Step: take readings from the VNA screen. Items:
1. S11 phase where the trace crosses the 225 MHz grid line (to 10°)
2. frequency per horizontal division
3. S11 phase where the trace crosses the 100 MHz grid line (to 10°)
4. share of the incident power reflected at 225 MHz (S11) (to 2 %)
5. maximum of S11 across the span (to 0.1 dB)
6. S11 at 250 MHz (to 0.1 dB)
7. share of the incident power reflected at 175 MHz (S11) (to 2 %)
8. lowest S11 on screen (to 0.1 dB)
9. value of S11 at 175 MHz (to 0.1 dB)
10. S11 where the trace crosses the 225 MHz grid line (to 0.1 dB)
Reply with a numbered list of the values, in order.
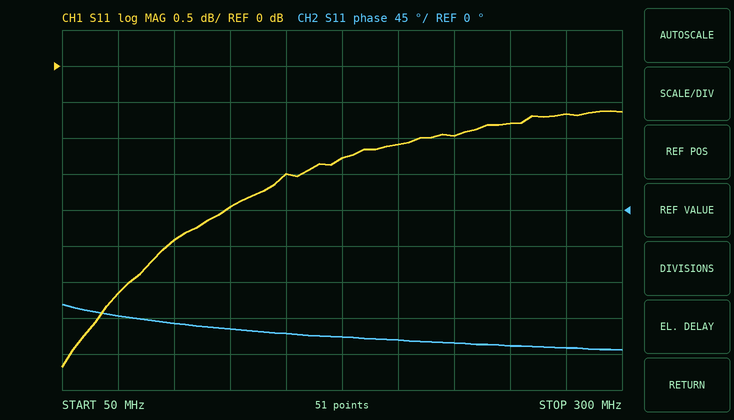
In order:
1. -170°
2. 25 MHz
3. -140°
4. 80 %
5. -0.6 dB
6. -0.8 dB
7. 74 %
8. -4.2 dB
9. -1.3 dB
10. -1.0 dB
